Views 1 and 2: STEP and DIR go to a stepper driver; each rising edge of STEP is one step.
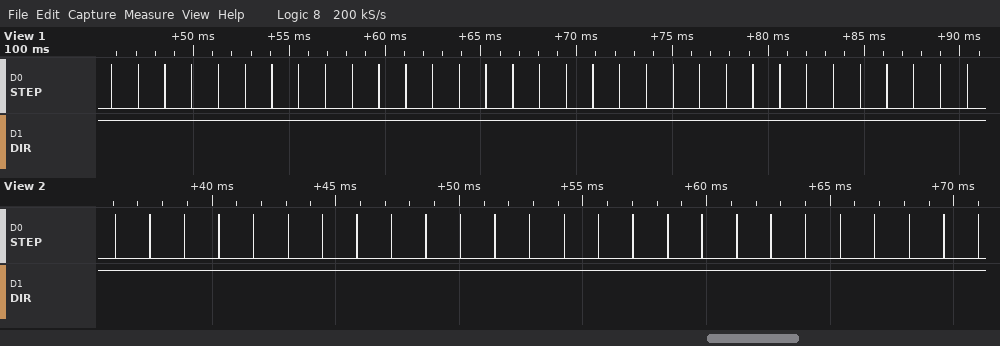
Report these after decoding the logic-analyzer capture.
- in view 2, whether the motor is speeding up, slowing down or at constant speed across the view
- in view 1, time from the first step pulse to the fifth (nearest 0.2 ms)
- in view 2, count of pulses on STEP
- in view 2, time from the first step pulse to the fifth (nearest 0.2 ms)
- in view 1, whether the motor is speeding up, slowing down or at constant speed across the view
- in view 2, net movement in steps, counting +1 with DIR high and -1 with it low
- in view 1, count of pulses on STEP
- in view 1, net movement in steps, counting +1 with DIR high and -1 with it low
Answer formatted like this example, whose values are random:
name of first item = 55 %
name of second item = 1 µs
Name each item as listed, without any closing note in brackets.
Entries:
in view 2, whether the motor is speeding up, slowing down or at constant speed across the view = constant speed
in view 1, time from the first step pulse to the fifth = 5.6 ms
in view 2, count of pulses on STEP = 26
in view 2, time from the first step pulse to the fifth = 5.6 ms
in view 1, whether the motor is speeding up, slowing down or at constant speed across the view = constant speed
in view 2, net movement in steps, counting +1 with DIR high and -1 with it low = +26
in view 1, count of pulses on STEP = 33
in view 1, net movement in steps, counting +1 with DIR high and -1 with it low = +33
